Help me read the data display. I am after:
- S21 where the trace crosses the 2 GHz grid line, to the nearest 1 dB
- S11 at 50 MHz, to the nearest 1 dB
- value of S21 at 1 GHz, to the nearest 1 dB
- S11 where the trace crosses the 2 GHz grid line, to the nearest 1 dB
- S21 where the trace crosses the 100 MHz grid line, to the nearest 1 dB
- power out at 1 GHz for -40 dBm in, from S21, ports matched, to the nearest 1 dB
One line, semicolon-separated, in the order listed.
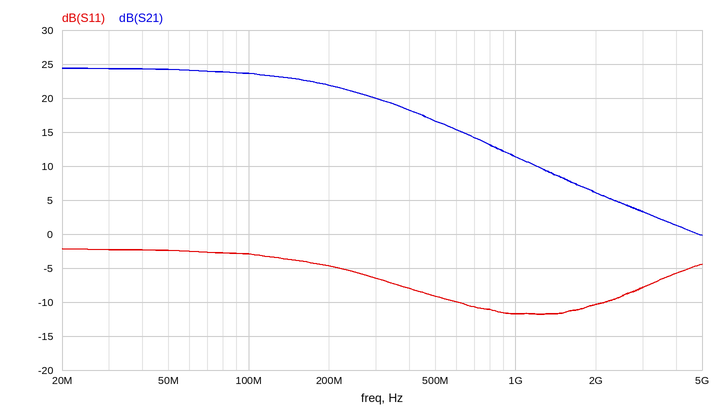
6 dB; -2 dB; 11 dB; -10 dB; 24 dB; -29 dBm
